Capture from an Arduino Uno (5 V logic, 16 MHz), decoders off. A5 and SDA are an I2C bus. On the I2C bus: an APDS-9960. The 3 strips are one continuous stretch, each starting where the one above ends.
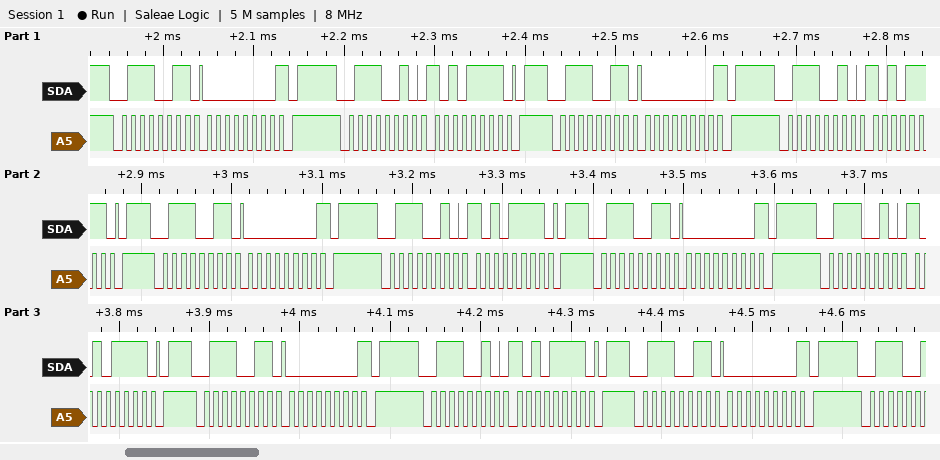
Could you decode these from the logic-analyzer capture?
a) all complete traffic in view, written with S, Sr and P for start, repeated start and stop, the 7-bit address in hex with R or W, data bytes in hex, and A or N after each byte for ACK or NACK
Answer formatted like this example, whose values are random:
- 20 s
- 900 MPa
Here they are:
- S 39R A 00 N P S 39W A AF A P S 39R A 00 N P S 39W A AF A P S 39R A 00 N P S 39W A AF A P S 39R A 00 N P S 39W A AF A P S 39R A 00 N P S 39W A AF A P S 39R A 00 N P
